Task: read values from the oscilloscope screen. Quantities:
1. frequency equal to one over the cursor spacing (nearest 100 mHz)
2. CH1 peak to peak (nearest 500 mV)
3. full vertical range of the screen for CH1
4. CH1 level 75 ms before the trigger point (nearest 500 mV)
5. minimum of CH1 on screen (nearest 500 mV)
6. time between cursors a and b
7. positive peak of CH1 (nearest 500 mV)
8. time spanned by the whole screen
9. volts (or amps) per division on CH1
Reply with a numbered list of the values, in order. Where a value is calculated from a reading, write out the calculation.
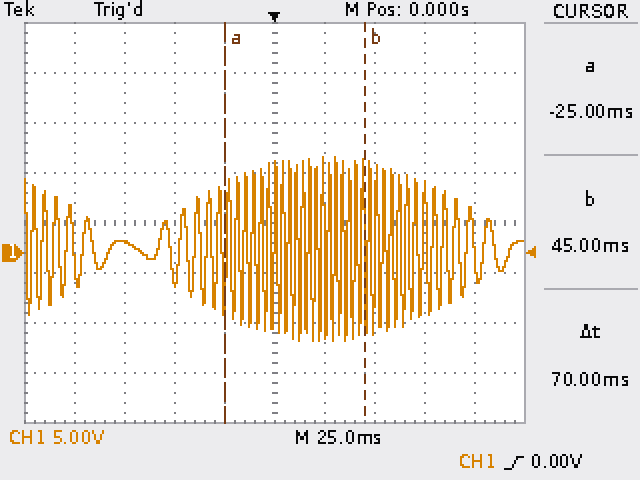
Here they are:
1. 1 / 70 ms ≈ 14.3 Hz
2. 9.5 V − (-9.0 V) = 18.5 V
3. 40 V
4. 1.0 V
5. -9.0 V
6. 70 ms
7. 9.5 V
8. 250 ms
9. 5 V
